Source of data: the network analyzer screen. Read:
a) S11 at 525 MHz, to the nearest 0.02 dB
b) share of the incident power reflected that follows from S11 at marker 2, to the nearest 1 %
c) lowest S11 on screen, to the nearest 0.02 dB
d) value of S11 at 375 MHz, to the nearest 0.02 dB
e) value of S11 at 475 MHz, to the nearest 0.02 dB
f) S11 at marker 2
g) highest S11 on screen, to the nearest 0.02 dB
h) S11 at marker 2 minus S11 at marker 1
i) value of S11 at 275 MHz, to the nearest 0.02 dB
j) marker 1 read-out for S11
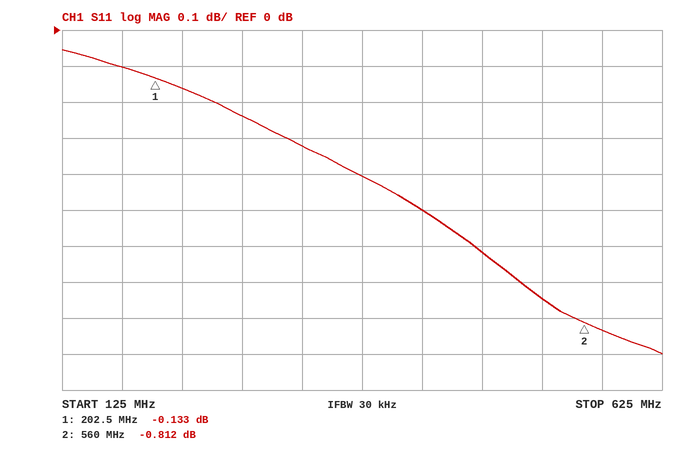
-0.74 dB
83 %
-0.90 dB
-0.40 dB
-0.62 dB
-0.812 dB
-0.06 dB
-0.679 dB
-0.24 dB
-0.133 dB
